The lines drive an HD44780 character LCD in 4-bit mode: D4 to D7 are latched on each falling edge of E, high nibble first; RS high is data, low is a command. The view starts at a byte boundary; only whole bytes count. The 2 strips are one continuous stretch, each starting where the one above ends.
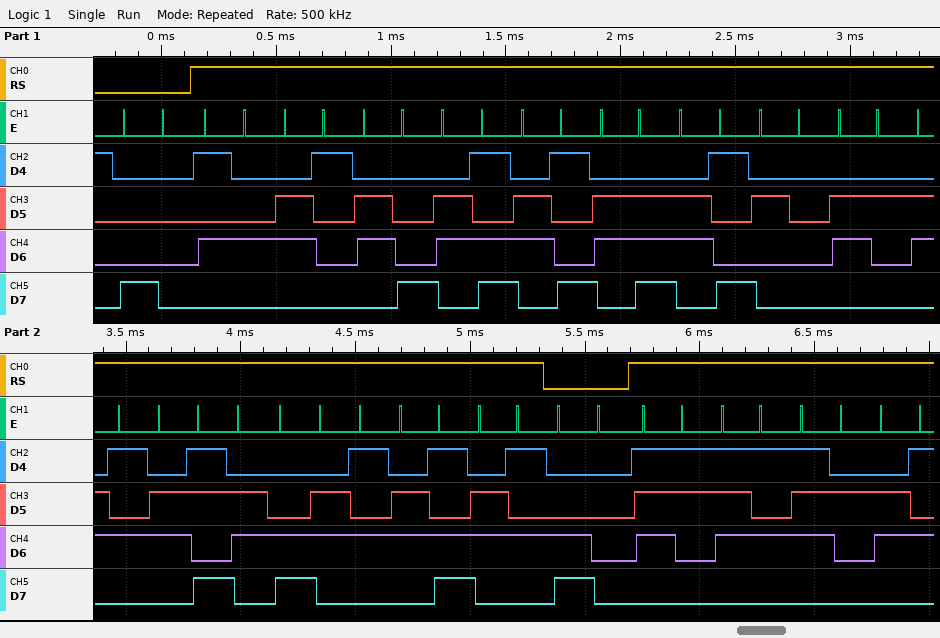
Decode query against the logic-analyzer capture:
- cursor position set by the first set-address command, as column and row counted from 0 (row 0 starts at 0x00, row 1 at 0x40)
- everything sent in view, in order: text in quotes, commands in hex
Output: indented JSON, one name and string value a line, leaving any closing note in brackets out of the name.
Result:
{
  "cursor position set by the first set-address command, as column and row counted from 0": "column 0, row 0",
  "everything sent in view, in order: text in quotes, commands in hex": "0x80 \"Tahmini bekleme\" 0xC0 \"sure\""
}
